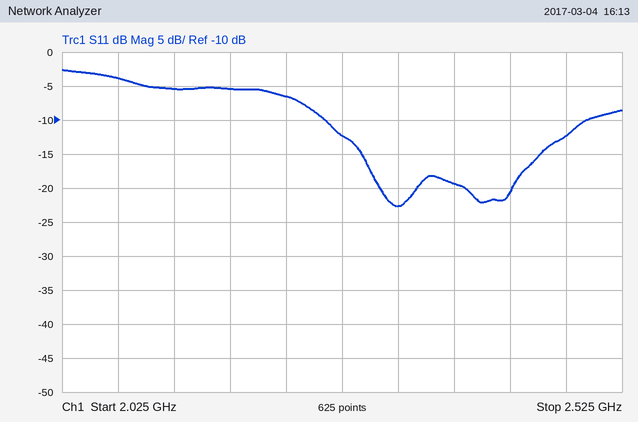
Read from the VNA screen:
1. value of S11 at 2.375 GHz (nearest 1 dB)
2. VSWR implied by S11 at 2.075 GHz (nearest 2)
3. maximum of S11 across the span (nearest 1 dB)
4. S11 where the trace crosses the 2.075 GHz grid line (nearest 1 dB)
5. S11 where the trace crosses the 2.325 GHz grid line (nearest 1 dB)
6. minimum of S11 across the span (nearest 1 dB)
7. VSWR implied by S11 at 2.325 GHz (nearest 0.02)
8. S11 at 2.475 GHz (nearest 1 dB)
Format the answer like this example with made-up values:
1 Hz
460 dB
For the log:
-19 dB
4
-3 dB
-4 dB
-23 dB
-23 dB
1.16
-12 dB
